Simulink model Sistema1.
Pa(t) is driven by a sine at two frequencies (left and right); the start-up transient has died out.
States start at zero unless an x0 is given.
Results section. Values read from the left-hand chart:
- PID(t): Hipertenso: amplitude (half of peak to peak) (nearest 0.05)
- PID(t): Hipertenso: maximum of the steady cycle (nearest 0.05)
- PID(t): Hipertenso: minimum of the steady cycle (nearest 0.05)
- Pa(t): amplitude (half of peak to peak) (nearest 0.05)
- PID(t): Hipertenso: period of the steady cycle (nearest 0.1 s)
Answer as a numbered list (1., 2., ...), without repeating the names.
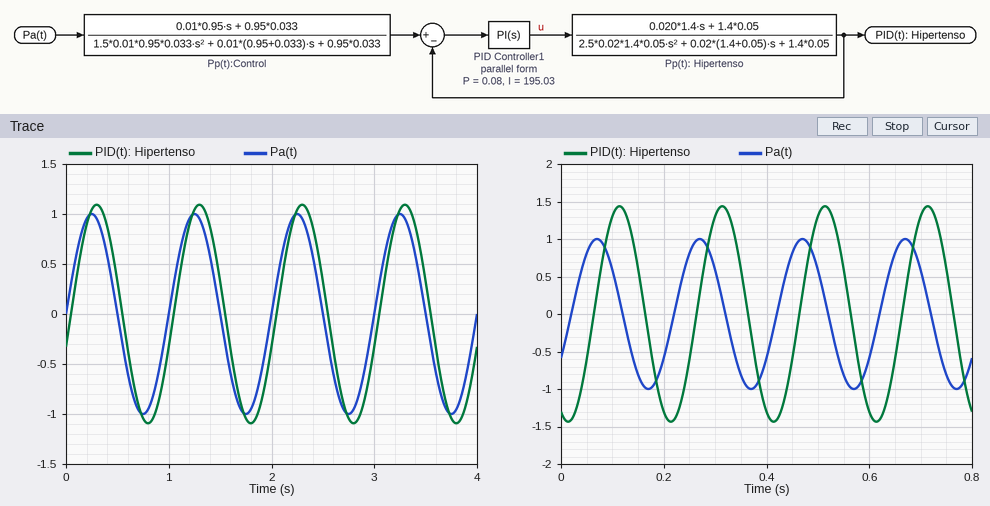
1. 1.10
2. 1.10
3. -1.10
4. 1.00
5. 1.0 s
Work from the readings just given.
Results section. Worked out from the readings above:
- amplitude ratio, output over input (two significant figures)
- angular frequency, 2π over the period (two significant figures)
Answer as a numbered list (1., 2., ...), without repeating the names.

1. 1.1
2. 6.3 rad/s
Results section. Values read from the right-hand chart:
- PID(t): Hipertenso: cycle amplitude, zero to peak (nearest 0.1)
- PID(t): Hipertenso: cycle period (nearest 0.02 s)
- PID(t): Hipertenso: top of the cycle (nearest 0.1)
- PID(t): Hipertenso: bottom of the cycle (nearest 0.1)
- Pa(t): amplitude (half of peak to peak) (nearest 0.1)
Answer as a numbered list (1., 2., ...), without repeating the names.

1. 1.4
2. 0.20 s
3. 1.4
4. -1.4
5. 1.0
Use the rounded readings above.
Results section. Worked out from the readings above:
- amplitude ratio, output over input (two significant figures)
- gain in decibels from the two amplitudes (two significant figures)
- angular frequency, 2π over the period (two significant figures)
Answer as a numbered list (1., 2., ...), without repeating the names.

1. 1.4
2. 2.9 dB
3. 31 rad/s
